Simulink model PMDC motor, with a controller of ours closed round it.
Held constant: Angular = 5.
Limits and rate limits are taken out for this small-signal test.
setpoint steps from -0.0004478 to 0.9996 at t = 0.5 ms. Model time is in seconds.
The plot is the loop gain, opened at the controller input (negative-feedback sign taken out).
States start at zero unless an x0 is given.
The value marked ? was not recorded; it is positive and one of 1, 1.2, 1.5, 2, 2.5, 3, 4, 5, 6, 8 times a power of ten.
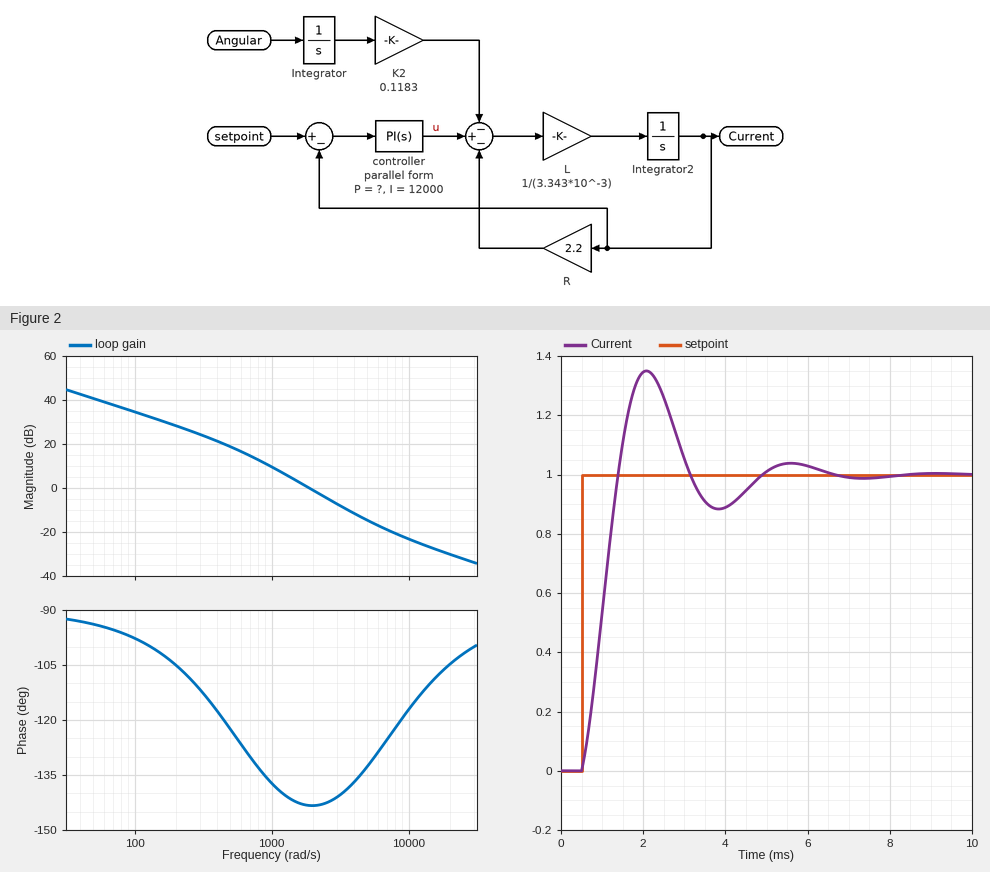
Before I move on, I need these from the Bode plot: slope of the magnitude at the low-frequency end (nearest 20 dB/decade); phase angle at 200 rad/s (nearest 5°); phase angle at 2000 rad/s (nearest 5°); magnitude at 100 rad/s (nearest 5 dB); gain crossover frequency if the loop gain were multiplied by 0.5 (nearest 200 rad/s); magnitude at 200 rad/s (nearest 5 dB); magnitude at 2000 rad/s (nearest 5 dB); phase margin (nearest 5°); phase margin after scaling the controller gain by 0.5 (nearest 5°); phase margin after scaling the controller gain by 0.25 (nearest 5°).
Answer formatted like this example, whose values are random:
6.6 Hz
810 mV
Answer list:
-20 dB/decade
-105°
-145°
35 dB
1200 rad/s
30 dB
0 dB
35°
40°
45°
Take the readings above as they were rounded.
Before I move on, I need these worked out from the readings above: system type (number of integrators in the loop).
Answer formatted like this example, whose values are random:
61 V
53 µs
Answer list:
1
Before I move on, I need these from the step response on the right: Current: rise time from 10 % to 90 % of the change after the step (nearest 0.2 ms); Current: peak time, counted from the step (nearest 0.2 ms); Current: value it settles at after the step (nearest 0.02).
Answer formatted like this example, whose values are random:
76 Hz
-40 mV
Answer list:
0.6 ms
1.6 ms
1.00
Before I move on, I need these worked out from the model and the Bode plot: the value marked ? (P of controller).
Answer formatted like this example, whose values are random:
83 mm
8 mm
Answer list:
2
